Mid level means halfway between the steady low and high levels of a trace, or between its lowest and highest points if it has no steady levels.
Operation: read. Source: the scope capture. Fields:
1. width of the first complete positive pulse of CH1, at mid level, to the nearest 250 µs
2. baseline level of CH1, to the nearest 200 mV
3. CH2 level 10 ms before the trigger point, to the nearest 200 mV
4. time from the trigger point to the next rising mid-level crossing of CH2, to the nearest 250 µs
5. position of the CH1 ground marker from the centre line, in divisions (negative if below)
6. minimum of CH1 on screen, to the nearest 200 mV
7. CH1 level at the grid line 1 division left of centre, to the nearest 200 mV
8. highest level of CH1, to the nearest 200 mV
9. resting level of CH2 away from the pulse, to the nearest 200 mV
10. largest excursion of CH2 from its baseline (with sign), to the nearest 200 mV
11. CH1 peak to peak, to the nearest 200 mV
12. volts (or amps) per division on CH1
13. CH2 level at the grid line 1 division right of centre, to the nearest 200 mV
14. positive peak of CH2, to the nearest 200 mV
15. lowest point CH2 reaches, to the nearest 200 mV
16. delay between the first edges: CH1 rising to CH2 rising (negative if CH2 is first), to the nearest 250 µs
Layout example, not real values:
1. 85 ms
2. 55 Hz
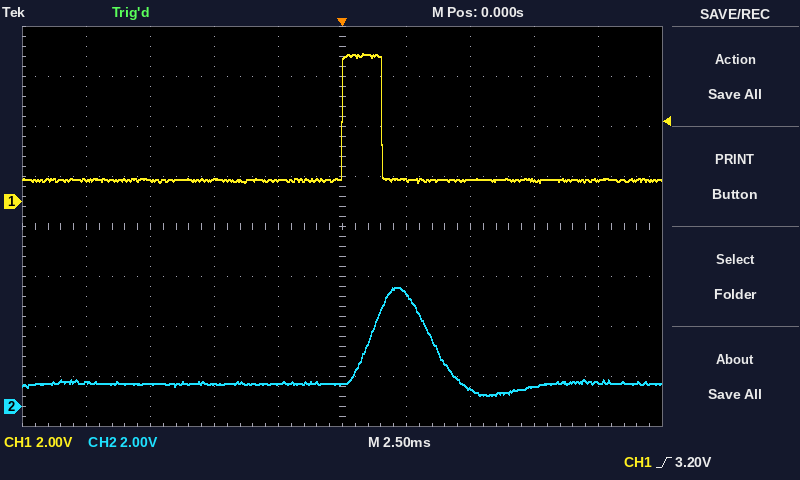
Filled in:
1. 1.50 ms
2. 800 mV
3. 1.0 V
4. 1.00 ms
5. +0.5 div
6. 800 mV
7. 800 mV
8. 6.0 V
9. 1.0 V
10. +3.8 V
11. 5.2 V
12. 2 V
13. 4.4 V
14. 4.8 V
15. 400 mV
16. +1.00 ms
